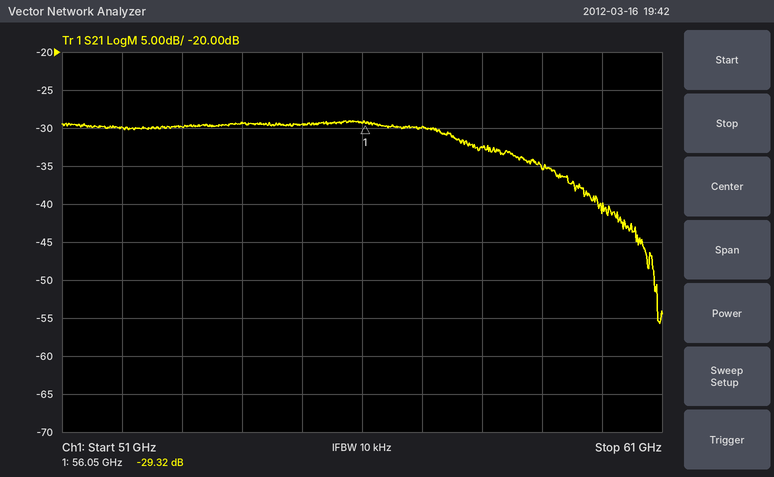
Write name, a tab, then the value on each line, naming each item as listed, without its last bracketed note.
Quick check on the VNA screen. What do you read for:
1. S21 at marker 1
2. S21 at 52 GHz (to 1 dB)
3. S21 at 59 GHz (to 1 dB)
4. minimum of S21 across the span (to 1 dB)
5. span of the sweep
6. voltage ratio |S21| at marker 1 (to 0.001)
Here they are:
S21 at marker 1	-29.32 dB
S21 at 52 GHz	-30 dB
S21 at 59 GHz	-35 dB
minimum of S21 across the span	-56 dB
span of the sweep	10 GHz
voltage ratio |S21| at marker 1	0.034
